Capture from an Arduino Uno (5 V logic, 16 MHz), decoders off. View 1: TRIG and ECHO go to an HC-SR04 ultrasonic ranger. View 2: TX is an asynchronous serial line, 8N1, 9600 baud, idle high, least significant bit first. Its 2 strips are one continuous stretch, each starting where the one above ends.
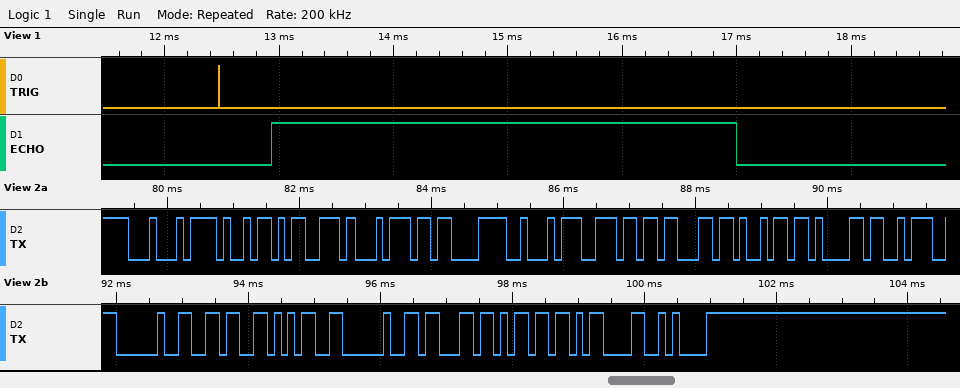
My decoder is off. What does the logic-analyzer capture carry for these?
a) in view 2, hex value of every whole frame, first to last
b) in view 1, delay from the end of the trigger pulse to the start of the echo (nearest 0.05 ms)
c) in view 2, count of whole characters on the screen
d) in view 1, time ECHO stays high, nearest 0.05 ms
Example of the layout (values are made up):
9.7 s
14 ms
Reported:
0x44 0x69 0x73 0x74 0xC3 0xA2 0x6E 0x63 0x69 0x61 0x3A 0x20 0x36 0x35 0x20 0x63 0x6D 0x0D 0x0A
0.45 ms
19
4.05 ms
